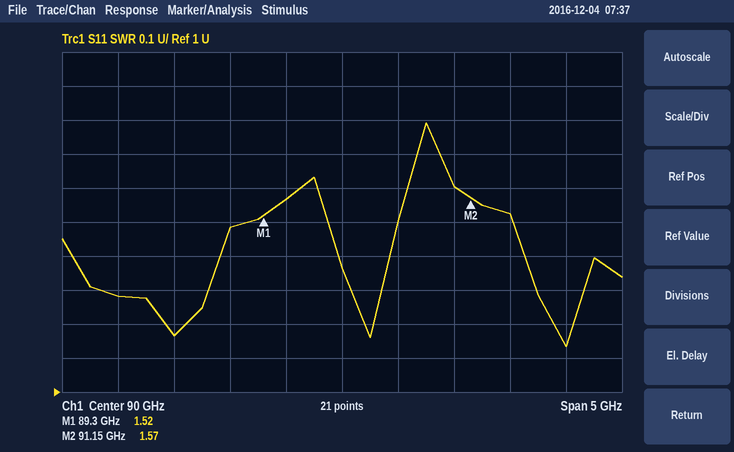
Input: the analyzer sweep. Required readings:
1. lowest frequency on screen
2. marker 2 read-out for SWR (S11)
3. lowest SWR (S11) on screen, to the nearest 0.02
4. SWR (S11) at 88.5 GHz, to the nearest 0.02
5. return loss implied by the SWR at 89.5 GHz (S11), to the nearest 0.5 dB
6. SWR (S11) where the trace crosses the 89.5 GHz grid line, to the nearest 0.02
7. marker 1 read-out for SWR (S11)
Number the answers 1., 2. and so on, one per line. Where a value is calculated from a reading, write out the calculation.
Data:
1. 87.5 GHz
2. 1.57
3. 1.14
4. 1.16
5. −20 log10((1.56 − 1)/(1.56 + 1)) ≈ 13.2 dB, so 13.0 dB to the nearest 0.5 dB
6. 1.56
7. 1.52
